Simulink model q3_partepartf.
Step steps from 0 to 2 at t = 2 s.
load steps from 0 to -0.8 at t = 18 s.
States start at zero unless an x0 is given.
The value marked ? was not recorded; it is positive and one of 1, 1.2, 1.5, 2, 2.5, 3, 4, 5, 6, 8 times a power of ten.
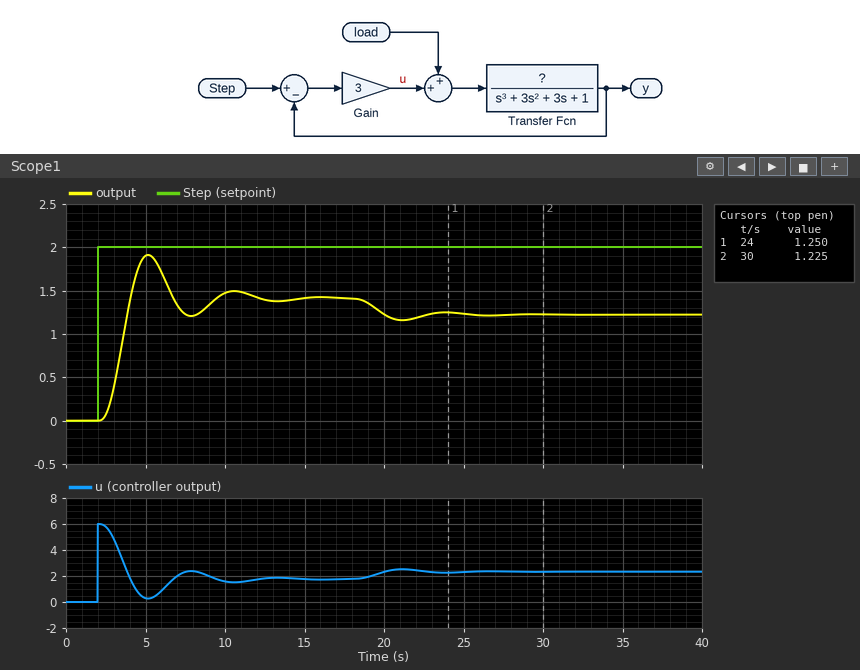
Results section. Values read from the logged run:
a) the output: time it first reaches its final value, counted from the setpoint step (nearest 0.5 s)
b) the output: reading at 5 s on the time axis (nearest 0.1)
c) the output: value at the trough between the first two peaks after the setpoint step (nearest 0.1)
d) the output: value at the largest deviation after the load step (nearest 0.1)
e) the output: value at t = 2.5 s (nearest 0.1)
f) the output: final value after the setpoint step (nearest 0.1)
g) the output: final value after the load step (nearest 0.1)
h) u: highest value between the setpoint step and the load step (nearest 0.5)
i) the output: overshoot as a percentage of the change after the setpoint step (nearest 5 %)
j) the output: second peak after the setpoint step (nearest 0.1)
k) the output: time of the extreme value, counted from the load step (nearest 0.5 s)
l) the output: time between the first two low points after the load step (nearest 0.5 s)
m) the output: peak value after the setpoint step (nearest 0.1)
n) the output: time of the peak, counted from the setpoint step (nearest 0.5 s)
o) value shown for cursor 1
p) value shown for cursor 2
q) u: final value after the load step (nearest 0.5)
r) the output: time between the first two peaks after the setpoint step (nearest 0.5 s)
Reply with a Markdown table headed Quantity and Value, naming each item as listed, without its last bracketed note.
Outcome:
| Quantity | Value |
|---|---|
| the output: time it first reaches its final value, counted from the setpoint step | 2.0 s |
| the output: reading at 5 s on the time axis | 1.9 |
| the output: value at the trough between the first two peaks after the setpoint step | 1.2 |
| the output: value at the largest deviation after the load step | 1.2 |
| the output: value at t = 2.5 s | 0.1 |
| the output: final value after the setpoint step | 1.4 |
| the output: final value after the load step | 1.2 |
| u: highest value between the setpoint step and the load step | 6.0 |
| the output: overshoot as a percentage of the change after the setpoint step | 35 % |
| the output: second peak after the setpoint step | 1.5 |
| the output: time of the extreme value, counted from the load step | 3.0 s |
| the output: time between the first two low points after the load step | 5.5 s |
| the output: peak value after the setpoint step | 1.9 |
| the output: time of the peak, counted from the setpoint step | 3.0 s |
| value shown for cursor 1 | 1.250 |
| value shown for cursor 2 | 1.225 |
| u: final value after the load step | 2.5 |
| the output: time between the first two peaks after the setpoint step | 5.5 s |
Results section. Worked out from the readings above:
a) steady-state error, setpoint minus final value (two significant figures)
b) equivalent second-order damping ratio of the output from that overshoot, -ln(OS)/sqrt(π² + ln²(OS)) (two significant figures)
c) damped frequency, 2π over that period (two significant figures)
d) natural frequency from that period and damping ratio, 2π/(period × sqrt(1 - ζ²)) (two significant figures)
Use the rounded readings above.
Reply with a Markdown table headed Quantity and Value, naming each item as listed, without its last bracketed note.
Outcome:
| Quantity | Value |
|---|---|
| steady-state error, setpoint minus final value | 0.60 |
| equivalent second-order damping ratio of the output from that overshoot, -ln(OS)/sqrt(π² + ln²(OS)) | 0.32 |
| damped frequency, 2π over that period | 1.1 rad/s |
| natural frequency from that period and damping ratio, 2π/(period × sqrt(1 - ζ²)) | 1.2 rad/s |
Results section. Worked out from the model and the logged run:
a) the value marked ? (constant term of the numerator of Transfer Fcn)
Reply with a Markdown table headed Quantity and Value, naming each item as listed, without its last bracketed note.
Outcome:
| Quantity | Value |
|---|---|
| the value marked ? | 0.8 |
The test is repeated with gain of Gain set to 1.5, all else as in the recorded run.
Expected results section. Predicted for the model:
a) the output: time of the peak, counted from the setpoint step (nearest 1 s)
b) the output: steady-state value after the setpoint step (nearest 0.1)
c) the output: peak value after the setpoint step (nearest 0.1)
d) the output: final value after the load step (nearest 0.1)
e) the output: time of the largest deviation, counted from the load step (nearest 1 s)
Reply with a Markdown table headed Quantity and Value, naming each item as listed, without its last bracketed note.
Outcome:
| Quantity | Value |
|---|---|
| the output: time of the peak, counted from the setpoint step | 4 s |
| the output: steady-state value after the setpoint step | 1.1 |
| the output: peak value after the setpoint step | 1.3 |
| the output: final value after the load step | 0.8 |
| the output: time of the largest deviation, counted from the load step | 4 s |
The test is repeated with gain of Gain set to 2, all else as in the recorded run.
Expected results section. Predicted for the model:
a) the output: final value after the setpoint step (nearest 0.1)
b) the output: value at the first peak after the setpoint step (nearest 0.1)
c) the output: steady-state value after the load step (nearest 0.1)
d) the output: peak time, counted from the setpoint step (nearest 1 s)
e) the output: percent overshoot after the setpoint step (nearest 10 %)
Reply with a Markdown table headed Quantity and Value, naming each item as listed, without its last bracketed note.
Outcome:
| Quantity | Value |
|---|---|
| the output: final value after the setpoint step | 1.2 |
| the output: value at the first peak after the setpoint step | 1.5 |
| the output: steady-state value after the load step | 1.0 |
| the output: peak time, counted from the setpoint step | 4 s |
| the output: percent overshoot after the setpoint step | 20 % |
